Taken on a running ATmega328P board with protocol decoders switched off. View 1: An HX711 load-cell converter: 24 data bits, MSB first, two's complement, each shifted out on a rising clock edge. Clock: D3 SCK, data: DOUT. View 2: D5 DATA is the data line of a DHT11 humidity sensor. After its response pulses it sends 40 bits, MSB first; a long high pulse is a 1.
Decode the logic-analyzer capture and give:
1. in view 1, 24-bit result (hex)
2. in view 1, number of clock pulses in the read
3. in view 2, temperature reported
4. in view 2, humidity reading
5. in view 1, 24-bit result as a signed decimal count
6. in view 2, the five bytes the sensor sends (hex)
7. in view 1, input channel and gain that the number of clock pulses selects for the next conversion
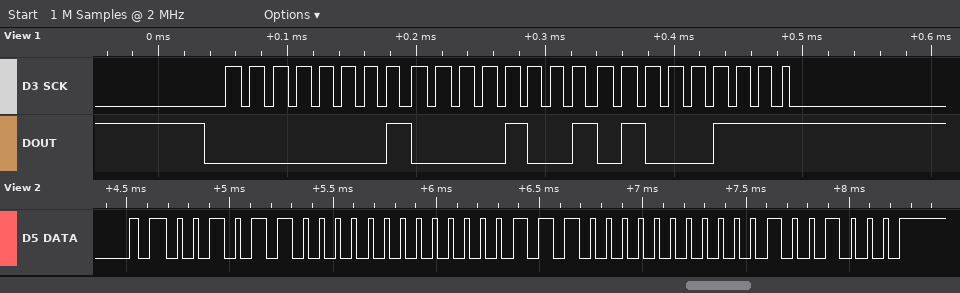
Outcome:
0x010947
25
28.0 °C
44 %
67911
2C 00 1C 00 48
channel A, gain 128
